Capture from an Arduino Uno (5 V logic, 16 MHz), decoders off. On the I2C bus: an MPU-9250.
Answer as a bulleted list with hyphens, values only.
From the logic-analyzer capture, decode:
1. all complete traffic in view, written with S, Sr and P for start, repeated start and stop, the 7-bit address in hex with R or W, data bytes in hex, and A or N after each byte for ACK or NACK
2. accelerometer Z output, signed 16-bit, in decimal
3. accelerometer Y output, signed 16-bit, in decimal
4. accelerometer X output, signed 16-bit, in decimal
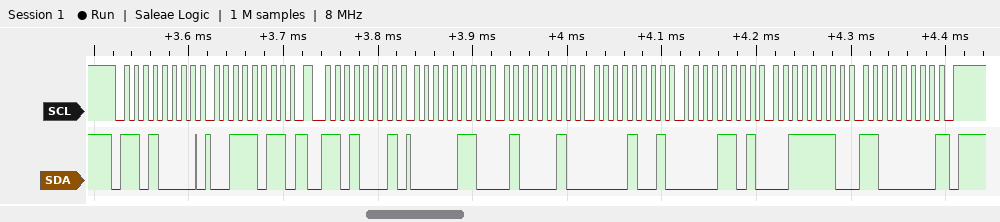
- S 68W A 3B A Sr 68R A 06 A 42 A 09 A 0D A 3E A C0 N P
- 16064
- 2317
- 1602
